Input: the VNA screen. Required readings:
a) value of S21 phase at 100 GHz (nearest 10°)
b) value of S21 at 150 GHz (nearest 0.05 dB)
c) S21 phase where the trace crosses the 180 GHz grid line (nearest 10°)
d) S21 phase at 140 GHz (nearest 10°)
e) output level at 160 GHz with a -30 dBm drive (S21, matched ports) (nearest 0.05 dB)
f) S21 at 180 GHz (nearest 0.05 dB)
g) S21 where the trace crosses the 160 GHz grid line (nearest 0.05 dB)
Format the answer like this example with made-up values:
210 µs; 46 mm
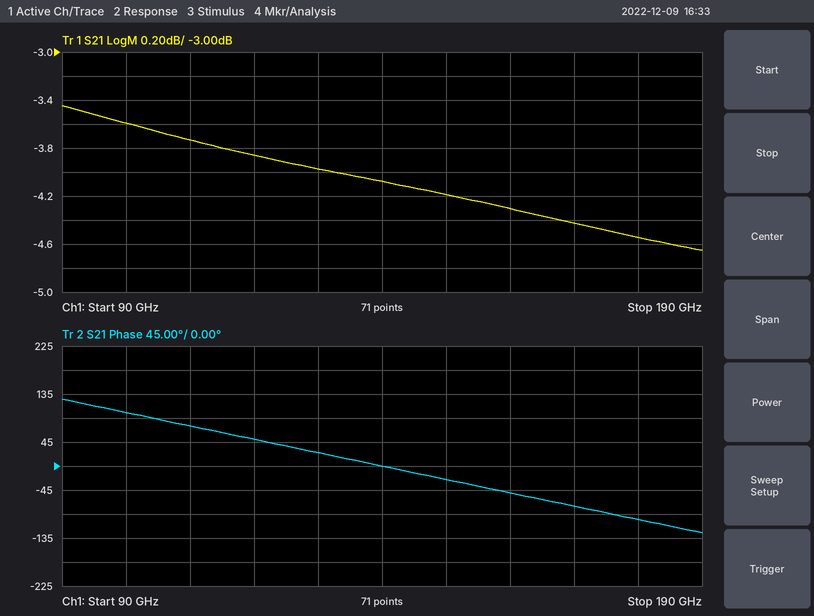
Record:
100°; -4.20 dB; -100°; 0°; -34.30 dBm; -4.55 dB; -4.30 dB
